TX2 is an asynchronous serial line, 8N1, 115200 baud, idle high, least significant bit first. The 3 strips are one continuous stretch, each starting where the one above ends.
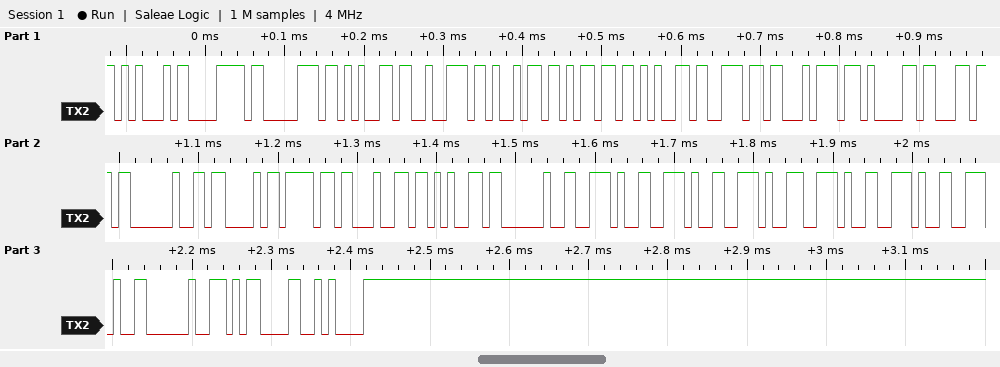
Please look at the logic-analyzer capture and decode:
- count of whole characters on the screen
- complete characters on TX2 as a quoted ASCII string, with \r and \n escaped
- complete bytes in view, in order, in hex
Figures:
27
"Experimental Code ...... \r\n"
45 78 70 65 72 69 6D 65 6E 74 61 6C 20 43 6F 64 65 20 2E 2E 2E 2E 2E 2E 20 0D 0A
